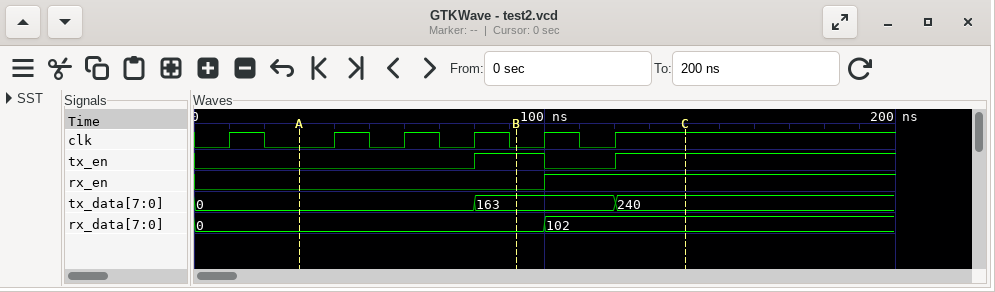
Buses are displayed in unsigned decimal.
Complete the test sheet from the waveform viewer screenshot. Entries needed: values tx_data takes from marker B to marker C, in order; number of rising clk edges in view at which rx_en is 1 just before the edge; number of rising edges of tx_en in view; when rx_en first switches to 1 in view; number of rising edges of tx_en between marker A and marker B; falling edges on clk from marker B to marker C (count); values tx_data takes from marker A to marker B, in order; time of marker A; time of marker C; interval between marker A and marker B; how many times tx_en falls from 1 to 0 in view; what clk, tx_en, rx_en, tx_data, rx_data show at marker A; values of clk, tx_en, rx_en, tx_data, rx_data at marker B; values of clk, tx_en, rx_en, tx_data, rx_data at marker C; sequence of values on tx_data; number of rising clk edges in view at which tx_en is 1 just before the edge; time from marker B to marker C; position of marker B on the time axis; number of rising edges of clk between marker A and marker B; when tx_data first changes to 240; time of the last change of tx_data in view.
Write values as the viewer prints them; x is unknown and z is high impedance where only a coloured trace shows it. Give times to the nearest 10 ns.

163, 240
1
2
100 ns
1
1
0, 163
30 ns
140 ns
60 ns
1
clk=0, tx_en=0, rx_en=0, tx_data=0, rx_data=0
clk=0, tx_en=1, rx_en=0, tx_data=163, rx_data=0
clk=1, tx_en=1, rx_en=1, tx_data=240, rx_data=102
0, 163, 240
1
50 ns
90 ns
3
120 ns
120 ns
